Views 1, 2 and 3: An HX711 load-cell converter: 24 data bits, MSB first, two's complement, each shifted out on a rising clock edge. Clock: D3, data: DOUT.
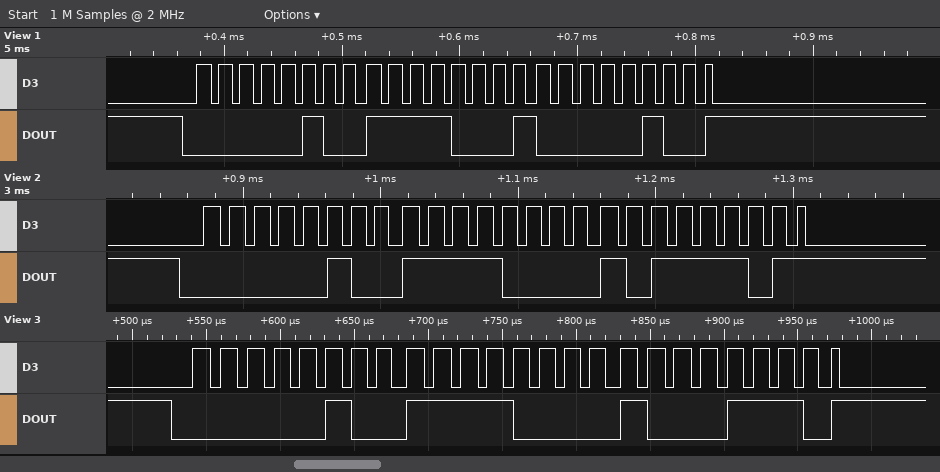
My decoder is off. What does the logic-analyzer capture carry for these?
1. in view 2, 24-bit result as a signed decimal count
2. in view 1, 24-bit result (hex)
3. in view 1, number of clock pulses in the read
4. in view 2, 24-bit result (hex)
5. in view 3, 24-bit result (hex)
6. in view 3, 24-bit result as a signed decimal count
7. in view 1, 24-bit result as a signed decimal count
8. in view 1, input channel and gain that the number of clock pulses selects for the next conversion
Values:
323773
0x04F104
25
0x04F0BD
0x04F08E
323726
323844
channel A, gain 128
